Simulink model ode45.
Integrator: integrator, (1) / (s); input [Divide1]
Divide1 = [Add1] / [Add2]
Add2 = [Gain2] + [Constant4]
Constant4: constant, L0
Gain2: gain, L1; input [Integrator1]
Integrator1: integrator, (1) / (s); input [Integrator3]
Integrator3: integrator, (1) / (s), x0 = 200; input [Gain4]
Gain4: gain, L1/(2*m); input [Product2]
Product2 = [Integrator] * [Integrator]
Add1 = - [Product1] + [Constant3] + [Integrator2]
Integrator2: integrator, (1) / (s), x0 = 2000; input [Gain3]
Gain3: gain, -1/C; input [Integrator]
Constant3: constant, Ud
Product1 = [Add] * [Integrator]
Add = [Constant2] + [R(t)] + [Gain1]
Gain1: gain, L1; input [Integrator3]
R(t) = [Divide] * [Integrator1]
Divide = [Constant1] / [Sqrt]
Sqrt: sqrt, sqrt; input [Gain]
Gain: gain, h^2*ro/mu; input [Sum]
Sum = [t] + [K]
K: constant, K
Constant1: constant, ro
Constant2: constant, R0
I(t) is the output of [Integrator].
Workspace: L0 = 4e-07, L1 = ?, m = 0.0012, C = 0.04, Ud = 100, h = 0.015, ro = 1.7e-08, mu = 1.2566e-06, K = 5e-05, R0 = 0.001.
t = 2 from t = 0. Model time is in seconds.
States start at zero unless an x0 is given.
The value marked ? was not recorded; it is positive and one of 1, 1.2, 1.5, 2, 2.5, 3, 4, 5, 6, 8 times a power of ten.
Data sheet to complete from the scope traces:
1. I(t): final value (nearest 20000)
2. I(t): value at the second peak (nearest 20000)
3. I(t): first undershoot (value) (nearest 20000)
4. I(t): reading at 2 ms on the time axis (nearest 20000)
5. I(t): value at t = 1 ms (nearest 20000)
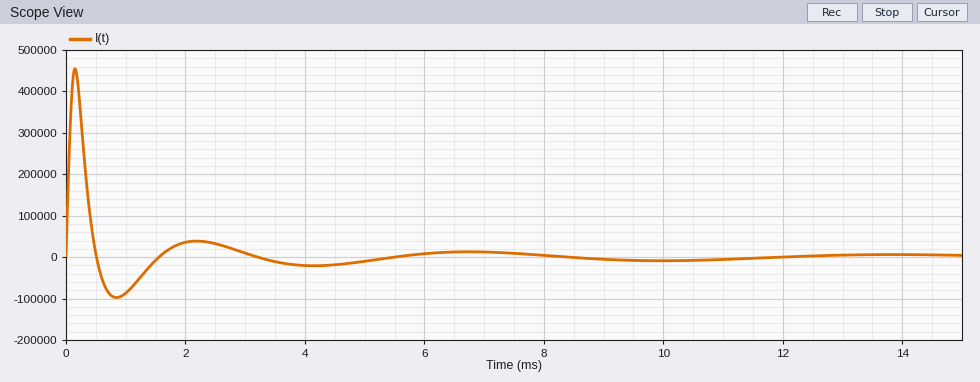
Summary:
0
40000
-100000
40000
-80000
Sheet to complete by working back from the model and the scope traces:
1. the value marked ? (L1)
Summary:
4e-07
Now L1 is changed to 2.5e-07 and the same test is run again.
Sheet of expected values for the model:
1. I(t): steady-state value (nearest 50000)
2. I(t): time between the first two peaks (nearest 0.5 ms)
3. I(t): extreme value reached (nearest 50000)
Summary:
0
1.5 ms
500000
